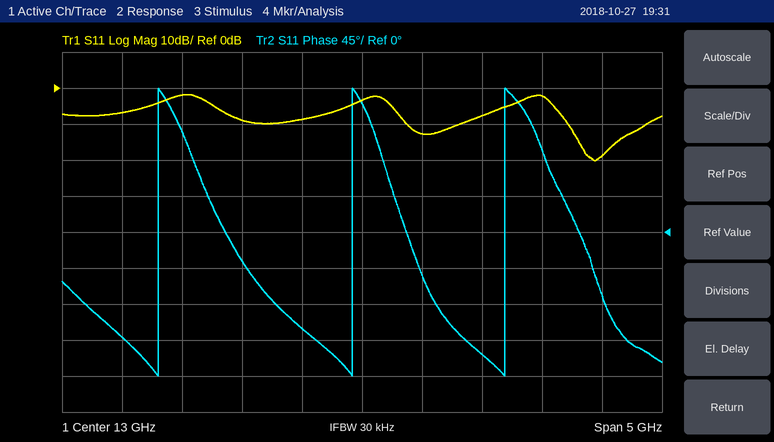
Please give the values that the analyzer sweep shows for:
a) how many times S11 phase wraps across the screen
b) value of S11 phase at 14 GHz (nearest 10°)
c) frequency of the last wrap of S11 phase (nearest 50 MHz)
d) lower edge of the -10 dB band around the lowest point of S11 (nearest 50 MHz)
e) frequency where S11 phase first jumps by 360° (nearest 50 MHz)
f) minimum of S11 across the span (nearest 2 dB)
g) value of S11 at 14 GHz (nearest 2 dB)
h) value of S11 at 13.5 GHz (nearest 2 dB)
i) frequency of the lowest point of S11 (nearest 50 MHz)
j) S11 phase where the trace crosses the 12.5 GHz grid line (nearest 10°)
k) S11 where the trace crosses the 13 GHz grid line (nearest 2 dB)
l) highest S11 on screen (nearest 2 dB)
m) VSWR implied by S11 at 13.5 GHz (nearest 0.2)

3
-150°
14.20 GHz
14.70 GHz
11.30 GHz
-20 dB
-8 dB
-12 dB
14.95 GHz
-120°
-4 dB
-2 dB
1.6
